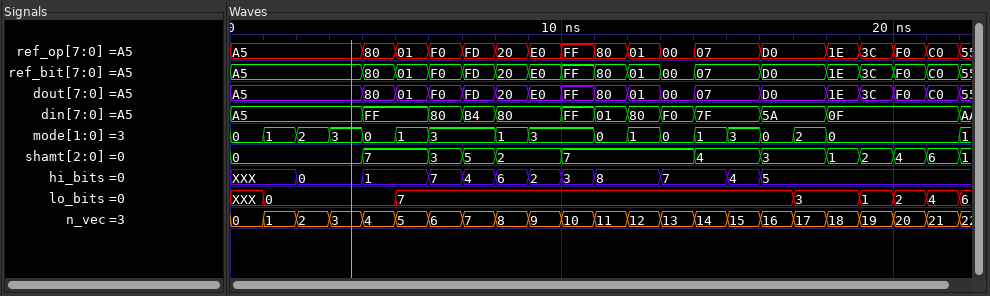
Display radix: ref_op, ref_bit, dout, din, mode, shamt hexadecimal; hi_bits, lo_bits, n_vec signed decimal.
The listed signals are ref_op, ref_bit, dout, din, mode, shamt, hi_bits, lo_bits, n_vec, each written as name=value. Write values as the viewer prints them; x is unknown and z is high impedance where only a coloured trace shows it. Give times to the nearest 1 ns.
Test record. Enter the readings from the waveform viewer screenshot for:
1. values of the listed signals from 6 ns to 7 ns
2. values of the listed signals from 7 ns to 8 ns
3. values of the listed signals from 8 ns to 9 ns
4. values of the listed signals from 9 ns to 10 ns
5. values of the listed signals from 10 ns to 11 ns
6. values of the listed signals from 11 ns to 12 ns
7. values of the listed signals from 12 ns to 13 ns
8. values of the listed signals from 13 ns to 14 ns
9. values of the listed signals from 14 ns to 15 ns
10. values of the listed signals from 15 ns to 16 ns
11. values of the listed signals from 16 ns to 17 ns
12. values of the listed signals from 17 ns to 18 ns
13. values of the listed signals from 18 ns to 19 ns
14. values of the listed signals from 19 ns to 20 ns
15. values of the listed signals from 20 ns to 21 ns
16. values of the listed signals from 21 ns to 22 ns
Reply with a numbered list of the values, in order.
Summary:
1. ref_op=F0, ref_bit=F0, dout=F0, din=80, mode=3, shamt=3, hi_bits=7, lo_bits=7, n_vec=6
2. ref_op=FD, ref_bit=FD, dout=FD, din=B4, mode=3, shamt=5, hi_bits=4, lo_bits=7, n_vec=7
3. ref_op=20, ref_bit=20, dout=20, din=80, mode=1, shamt=2, hi_bits=6, lo_bits=7, n_vec=8
4. ref_op=E0, ref_bit=E0, dout=E0, din=80, mode=3, shamt=2, hi_bits=2, lo_bits=7, n_vec=9
5. ref_op=FF, ref_bit=FF, dout=FF, din=FF, mode=3, shamt=7, hi_bits=3, lo_bits=7, n_vec=10
6. ref_op=80, ref_bit=80, dout=80, din=01, mode=0, shamt=7, hi_bits=8, lo_bits=7, n_vec=11
7. ref_op=01, ref_bit=01, dout=01, din=80, mode=1, shamt=7, hi_bits=8, lo_bits=7, n_vec=12
8. ref_op=00, ref_bit=00, dout=00, din=F0, mode=0, shamt=7, hi_bits=7, lo_bits=7, n_vec=13
9. ref_op=07, ref_bit=07, dout=07, din=7F, mode=1, shamt=4, hi_bits=7, lo_bits=7, n_vec=14
10. ref_op=07, ref_bit=07, dout=07, din=7F, mode=3, shamt=4, hi_bits=4, lo_bits=7, n_vec=15
11. ref_op=D0, ref_bit=D0, dout=D0, din=5A, mode=0, shamt=3, hi_bits=5, lo_bits=7, n_vec=16
12. ref_op=D0, ref_bit=D0, dout=D0, din=5A, mode=2, shamt=3, hi_bits=5, lo_bits=3, n_vec=17
13. ref_op=1E, ref_bit=1E, dout=1E, din=0F, mode=0, shamt=1, hi_bits=5, lo_bits=3, n_vec=18
14. ref_op=3C, ref_bit=3C, dout=3C, din=0F, mode=0, shamt=2, hi_bits=5, lo_bits=1, n_vec=19
15. ref_op=F0, ref_bit=F0, dout=F0, din=0F, mode=0, shamt=4, hi_bits=5, lo_bits=2, n_vec=20
16. ref_op=C0, ref_bit=C0, dout=C0, din=0F, mode=0, shamt=6, hi_bits=5, lo_bits=4, n_vec=21
